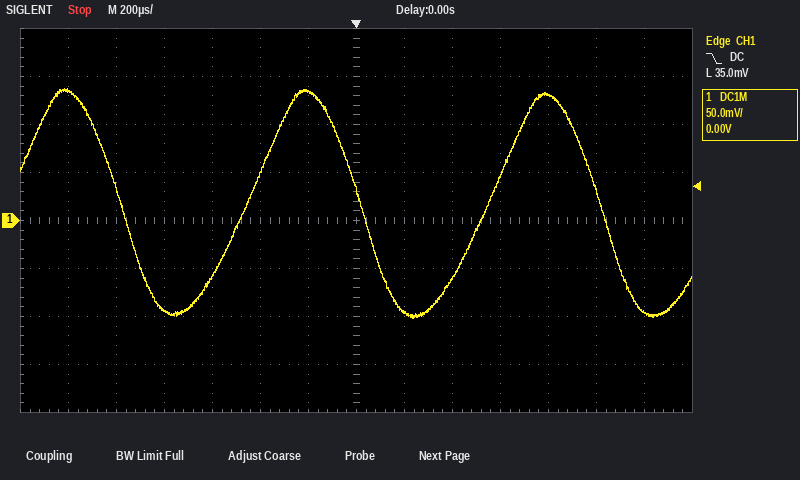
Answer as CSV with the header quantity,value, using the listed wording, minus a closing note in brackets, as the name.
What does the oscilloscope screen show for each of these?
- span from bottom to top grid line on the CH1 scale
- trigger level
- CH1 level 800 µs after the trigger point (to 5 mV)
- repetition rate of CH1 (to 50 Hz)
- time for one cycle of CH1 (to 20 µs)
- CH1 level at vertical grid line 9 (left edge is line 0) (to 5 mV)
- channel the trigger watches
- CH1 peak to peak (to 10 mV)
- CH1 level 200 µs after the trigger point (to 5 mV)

quantity,value
span from bottom to top grid line on the CH1 scale,400 mV
trigger level,35.0 mV
CH1 level 800 µs after the trigger point,130 mV
repetition rate of CH1,1.00 kHz
time for one cycle of CH1,1.00 ms
CH1 level at vertical grid line 9 (left edge is line 0),-60 mV
channel the trigger watches,CH1
CH1 peak to peak,240 mV
CH1 level 200 µs after the trigger point,-95 mV
